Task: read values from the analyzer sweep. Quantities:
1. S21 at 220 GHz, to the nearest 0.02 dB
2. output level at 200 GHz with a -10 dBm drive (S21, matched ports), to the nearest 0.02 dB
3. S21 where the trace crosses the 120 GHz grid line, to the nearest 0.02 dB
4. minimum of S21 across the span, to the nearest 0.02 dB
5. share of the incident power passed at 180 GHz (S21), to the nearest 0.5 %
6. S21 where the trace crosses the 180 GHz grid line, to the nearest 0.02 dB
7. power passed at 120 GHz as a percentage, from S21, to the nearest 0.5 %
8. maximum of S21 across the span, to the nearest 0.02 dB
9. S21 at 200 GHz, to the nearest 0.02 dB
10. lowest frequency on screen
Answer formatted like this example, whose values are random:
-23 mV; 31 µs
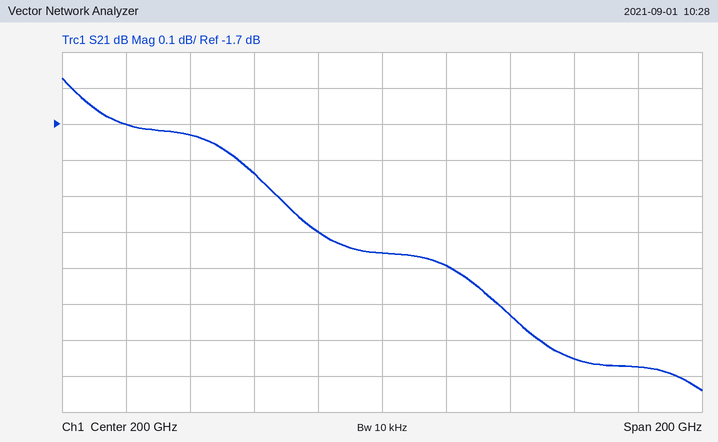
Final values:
-2.10 dB; -12.06 dBm; -1.70 dB; -2.44 dB; 63.0 %; -2.00 dB; 67.5 %; -1.58 dB; -2.06 dB; 100 GHz
